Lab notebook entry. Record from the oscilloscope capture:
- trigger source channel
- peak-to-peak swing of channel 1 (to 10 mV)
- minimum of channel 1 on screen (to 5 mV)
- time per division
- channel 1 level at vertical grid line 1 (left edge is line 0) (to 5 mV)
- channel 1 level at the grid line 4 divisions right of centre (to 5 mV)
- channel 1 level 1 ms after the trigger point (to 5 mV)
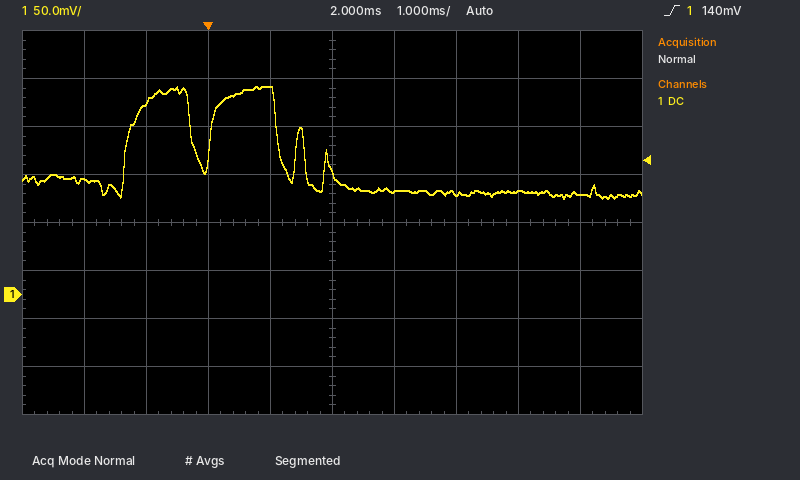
channel 1
120 mV
100 mV
1 ms
120 mV
105 mV
215 mV
